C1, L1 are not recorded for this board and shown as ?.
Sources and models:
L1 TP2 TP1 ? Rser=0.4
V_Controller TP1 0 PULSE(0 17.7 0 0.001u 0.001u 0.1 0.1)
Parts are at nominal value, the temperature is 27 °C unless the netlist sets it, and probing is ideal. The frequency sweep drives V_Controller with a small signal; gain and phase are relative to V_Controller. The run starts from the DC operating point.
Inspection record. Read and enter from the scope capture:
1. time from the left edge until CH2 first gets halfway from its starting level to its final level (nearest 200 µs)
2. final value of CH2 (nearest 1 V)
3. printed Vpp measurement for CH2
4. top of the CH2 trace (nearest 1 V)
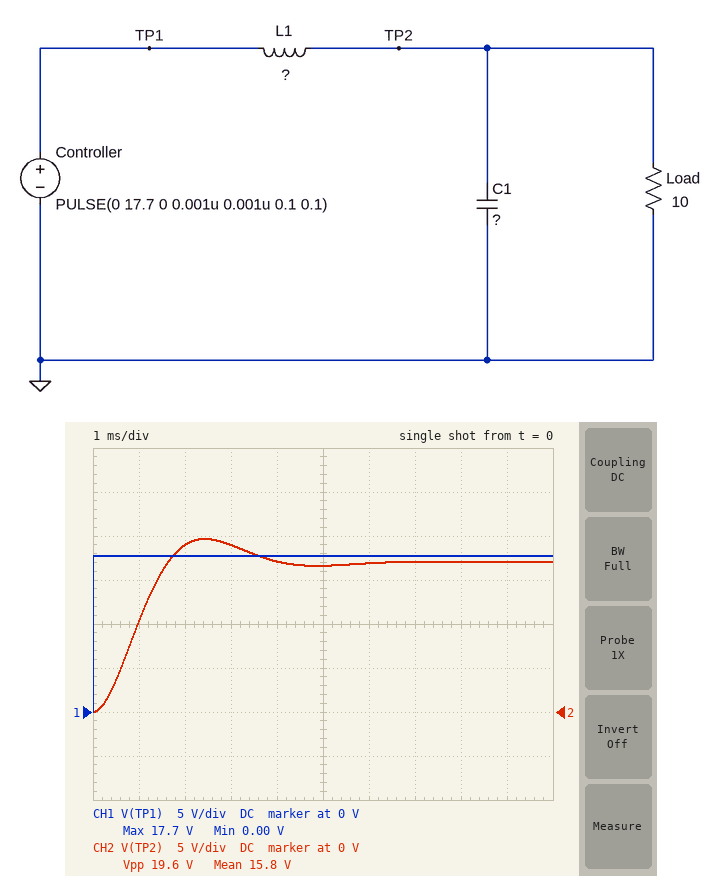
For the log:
800 µs
17 V
19.6 V
20 V
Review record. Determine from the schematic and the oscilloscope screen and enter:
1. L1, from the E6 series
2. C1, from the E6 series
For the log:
6.8 mH
68 µF
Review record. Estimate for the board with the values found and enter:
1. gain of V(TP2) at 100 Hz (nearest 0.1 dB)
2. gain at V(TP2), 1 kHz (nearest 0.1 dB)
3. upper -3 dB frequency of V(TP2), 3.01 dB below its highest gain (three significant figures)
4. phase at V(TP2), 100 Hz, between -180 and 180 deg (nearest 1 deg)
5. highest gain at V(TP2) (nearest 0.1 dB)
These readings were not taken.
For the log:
0.3 dB
-25.0 dB
278 Hz
-27 deg
0.8 dB
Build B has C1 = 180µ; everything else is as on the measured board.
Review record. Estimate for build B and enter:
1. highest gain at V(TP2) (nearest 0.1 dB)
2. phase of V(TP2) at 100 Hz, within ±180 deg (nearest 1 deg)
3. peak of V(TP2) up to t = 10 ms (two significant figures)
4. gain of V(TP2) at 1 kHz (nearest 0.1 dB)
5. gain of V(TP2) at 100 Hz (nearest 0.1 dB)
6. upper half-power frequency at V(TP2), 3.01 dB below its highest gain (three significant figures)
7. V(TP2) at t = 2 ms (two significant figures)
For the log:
3.7 dB
-40 deg
23 V
-33.5 dB
2.7 dB
174 Hz
15 V
